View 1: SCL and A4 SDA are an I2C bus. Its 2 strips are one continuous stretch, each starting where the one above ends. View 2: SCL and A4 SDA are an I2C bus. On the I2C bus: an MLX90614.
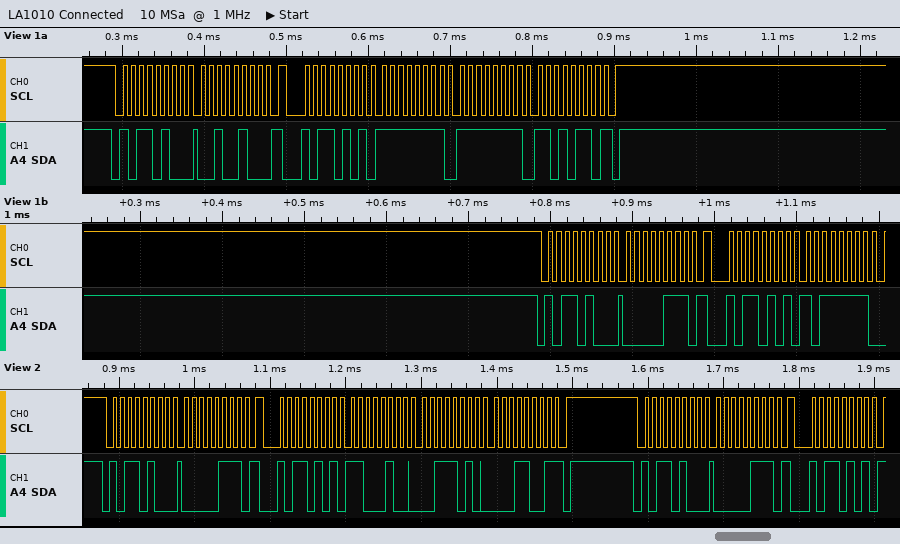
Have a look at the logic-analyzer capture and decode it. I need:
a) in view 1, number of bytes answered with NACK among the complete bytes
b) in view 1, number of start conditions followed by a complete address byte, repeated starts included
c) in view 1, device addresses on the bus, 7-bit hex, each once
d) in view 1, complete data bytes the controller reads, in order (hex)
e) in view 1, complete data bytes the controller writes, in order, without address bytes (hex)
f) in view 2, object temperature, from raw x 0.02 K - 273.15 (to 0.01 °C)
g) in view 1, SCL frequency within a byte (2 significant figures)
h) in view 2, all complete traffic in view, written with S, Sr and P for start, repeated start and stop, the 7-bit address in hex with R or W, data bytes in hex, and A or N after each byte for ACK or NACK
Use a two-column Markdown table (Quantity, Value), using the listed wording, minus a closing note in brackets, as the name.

| Quantity | Value |
|---|---|
| in view 1, number of bytes answered with NACK among the complete bytes | 1 |
| in view 1, number of start conditions followed by a complete address byte, repeated starts included | 4 |
| in view 1, device addresses on the bus, 7-bit hex, each once | 0x5A |
| in view 1, complete data bytes the controller reads, in order | FF FF D6 BF |
| in view 1, complete data bytes the controller writes, in order, without address bytes | 24 07 |
| in view 2, object temperature, from raw x 0.02 K - 273.15 | 27.73 °C |
| in view 1, SCL frequency within a byte | 100 kHz |
| in view 2, all complete traffic in view, written with S, Sr and P for start, repeated start and stop, the 7-bit address in hex with R or W, data bytes in hex, and A or N after each byte for ACK or NACK | S 5AW A 07 A Sr 5AR A C4 A 3A A 19 N P S 5AW A 07 A Sr 5AR A |
